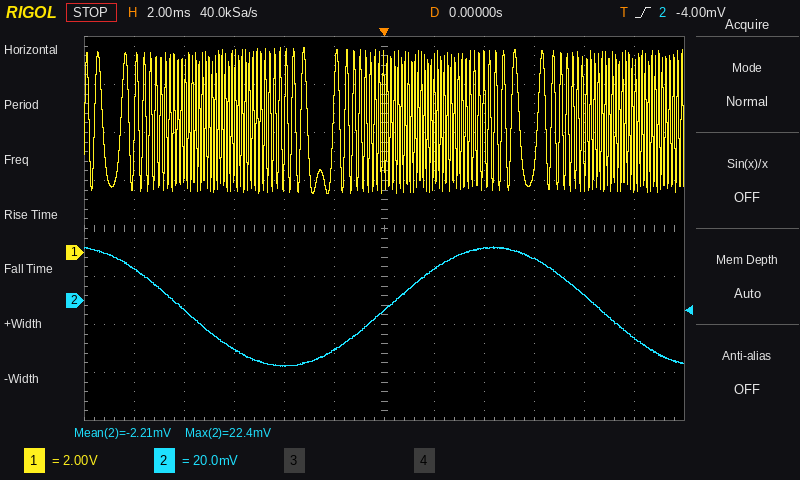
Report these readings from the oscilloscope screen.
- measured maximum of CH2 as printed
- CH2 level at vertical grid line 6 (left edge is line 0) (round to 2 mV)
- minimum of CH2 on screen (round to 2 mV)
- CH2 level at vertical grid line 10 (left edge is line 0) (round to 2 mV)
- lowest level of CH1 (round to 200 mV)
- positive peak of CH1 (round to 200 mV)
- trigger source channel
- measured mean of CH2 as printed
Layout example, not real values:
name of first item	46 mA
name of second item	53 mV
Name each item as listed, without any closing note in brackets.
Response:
measured maximum of CH2 as printed	22.4 mV
CH2 level at vertical grid line 6 (left edge is line 0)	-4 mV
minimum of CH2 on screen	-28 mV
CH2 level at vertical grid line 10 (left edge is line 0)	2 mV
lowest level of CH1	2.4 V
positive peak of CH1	8.6 V
trigger source channel	CH2
measured mean of CH2 as printed	-2.21 mV
